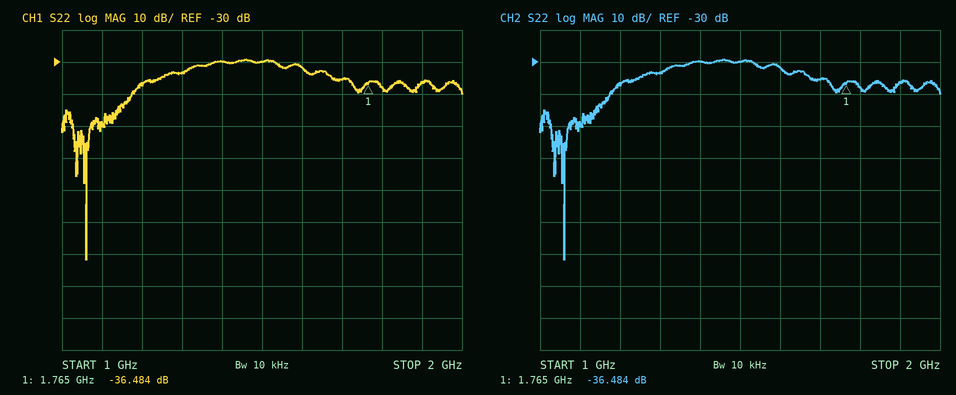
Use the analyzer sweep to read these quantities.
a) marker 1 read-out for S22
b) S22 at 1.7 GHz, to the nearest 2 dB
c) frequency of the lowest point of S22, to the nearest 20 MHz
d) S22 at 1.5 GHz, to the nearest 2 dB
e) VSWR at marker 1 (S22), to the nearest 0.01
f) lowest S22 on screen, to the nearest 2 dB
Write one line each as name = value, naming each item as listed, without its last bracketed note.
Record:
marker 1 read-out for S22 = -36.484 dB
S22 at 1.7 GHz, to the nearest 2 dB = -36 dB
frequency of the lowest point of S22, to the nearest 20 MHz = 1.06 GHz
S22 at 1.5 GHz, to the nearest 2 dB = -30 dB
VSWR at marker 1 (S22), to the nearest 0.01 = 1.03
lowest S22 on screen, to the nearest 2 dB = -92 dB
